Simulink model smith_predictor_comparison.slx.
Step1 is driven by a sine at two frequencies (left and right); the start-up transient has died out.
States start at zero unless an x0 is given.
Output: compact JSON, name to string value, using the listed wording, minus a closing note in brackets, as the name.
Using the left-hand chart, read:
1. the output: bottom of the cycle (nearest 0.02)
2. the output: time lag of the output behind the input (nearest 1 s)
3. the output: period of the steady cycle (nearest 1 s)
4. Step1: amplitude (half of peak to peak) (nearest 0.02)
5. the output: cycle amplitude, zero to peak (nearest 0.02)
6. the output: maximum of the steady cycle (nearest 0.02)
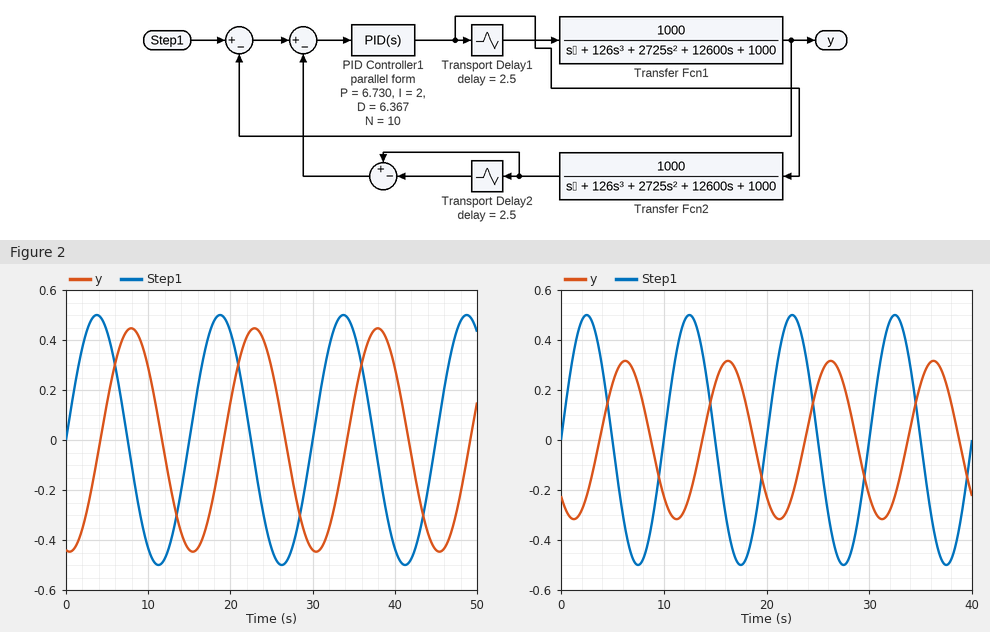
{"the output: bottom of the cycle": "-0.44", "the output: time lag of the output behind the input": "4 s", "the output: period of the steady cycle": "15 s", "Step1: amplitude (half of peak to peak)": "0.50", "the output: cycle amplitude, zero to peak": "0.44", "the output: maximum of the steady cycle": "0.44"}
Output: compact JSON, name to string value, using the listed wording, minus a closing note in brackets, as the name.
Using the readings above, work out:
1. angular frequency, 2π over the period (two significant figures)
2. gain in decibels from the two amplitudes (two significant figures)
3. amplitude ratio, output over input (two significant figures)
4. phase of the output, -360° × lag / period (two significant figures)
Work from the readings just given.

{"angular frequency, 2π over the period": "0.42 rad/s", "gain in decibels from the two amplitudes": "-1.1 dB", "amplitude ratio, output over input": "0.88", "phase of the output, -360° × lag / period": "-96°"}
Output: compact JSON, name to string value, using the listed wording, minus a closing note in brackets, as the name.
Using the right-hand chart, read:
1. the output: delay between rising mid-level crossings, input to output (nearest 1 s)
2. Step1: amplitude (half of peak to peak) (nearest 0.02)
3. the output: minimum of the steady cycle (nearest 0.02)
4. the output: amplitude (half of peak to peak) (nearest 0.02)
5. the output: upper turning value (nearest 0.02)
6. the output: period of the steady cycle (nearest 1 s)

{"the output: delay between rising mid-level crossings, input to output": "4 s", "Step1: amplitude (half of peak to peak)": "0.50", "the output: minimum of the steady cycle": "-0.32", "the output: amplitude (half of peak to peak)": "0.32", "the output: upper turning value": "0.32", "the output: period of the steady cycle": "10 s"}
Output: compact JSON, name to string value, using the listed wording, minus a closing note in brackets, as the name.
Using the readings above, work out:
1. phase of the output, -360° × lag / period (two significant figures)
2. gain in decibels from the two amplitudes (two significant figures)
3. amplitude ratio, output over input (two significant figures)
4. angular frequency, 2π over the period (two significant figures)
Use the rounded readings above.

{"phase of the output, -360° × lag / period": "-140°", "gain in decibels from the two amplitudes": "-3.9 dB", "amplitude ratio, output over input": "0.64", "angular frequency, 2π over the period": "0.63 rad/s"}
